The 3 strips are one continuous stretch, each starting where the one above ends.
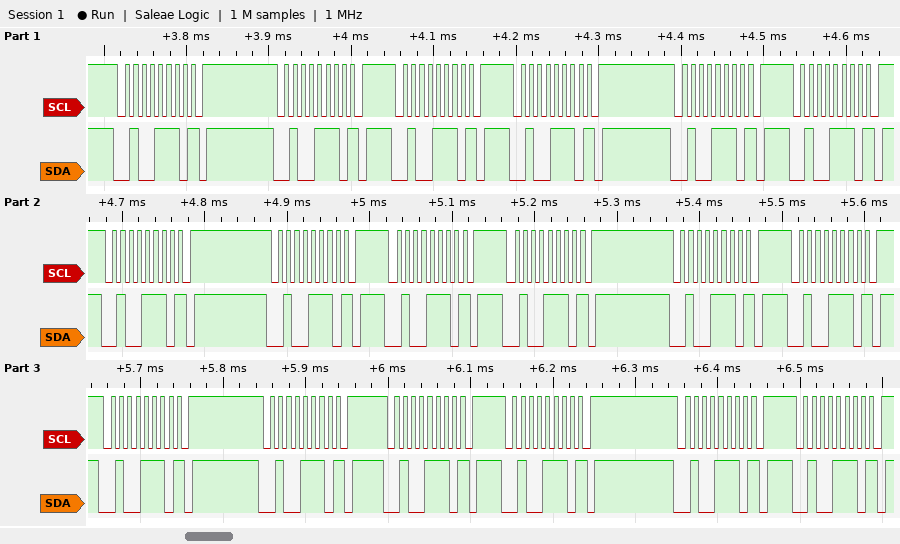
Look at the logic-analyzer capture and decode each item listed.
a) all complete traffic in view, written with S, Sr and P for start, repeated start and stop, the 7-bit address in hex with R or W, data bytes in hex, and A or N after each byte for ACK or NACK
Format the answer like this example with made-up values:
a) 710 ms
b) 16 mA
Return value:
a) S 27W N P S 27W N P S 27W N P S 27W N P S 27W N P S 27W N P S 27W N P S 27W N P S 27W N P S 27W N P S 27W N P S 27W N P S 27W N P S 27W N P S 27W N P S 27W N P S 27W N P S 27W N P
